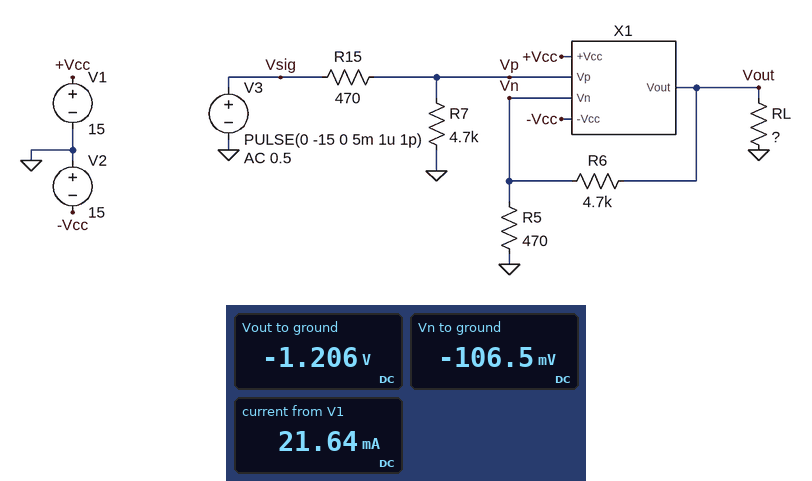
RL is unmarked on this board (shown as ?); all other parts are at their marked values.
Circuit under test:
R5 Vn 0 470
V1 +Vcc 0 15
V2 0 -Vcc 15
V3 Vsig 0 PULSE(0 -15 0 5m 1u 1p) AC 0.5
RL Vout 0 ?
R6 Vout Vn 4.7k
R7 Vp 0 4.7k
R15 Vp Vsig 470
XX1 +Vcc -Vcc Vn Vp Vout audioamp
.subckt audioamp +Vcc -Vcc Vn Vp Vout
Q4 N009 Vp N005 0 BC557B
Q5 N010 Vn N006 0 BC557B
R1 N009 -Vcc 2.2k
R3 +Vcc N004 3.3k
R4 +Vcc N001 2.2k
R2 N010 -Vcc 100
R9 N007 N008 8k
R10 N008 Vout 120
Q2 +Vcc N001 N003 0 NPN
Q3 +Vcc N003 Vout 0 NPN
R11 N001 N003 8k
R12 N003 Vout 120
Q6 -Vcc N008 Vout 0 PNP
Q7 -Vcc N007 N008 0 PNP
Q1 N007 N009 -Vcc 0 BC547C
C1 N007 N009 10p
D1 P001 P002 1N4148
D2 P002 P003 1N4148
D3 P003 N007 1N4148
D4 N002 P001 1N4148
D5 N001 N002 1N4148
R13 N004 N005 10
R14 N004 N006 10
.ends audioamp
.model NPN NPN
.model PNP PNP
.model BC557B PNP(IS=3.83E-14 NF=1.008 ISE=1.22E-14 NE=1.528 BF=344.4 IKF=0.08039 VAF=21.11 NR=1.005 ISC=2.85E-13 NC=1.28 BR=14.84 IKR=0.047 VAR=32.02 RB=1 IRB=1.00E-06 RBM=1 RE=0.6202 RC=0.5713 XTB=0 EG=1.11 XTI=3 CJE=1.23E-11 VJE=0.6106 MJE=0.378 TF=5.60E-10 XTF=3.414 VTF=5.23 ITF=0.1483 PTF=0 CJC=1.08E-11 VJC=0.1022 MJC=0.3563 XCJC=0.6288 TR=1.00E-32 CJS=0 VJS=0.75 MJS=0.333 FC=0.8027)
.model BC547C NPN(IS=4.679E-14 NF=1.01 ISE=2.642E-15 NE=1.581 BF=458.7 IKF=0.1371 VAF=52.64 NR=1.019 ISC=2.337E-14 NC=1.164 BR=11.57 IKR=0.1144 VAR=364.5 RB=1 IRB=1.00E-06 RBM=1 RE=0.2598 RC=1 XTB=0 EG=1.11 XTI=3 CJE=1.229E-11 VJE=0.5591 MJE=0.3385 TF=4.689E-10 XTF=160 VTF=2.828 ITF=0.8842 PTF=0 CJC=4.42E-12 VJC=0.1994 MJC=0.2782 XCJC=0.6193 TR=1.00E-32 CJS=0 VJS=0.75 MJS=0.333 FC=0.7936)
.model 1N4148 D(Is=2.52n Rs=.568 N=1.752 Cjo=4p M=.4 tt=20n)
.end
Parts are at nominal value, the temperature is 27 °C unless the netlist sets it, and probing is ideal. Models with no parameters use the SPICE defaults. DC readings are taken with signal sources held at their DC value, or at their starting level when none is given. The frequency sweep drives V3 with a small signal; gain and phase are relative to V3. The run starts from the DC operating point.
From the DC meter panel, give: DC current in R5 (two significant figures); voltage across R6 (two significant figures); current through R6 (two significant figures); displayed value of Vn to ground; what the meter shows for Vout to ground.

230 µA
1.1 V
230 µA
-106.5 mV
-1.206 V
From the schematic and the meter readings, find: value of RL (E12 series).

10 Ω
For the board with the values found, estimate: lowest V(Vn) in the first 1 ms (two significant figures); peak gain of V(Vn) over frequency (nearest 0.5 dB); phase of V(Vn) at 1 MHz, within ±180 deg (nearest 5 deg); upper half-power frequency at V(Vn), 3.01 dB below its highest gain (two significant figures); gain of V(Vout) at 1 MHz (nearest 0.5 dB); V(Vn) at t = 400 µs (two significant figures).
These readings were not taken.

-1.2 V
0 dB
-5 deg
11 MHz
20.0 dB
-1.2 V
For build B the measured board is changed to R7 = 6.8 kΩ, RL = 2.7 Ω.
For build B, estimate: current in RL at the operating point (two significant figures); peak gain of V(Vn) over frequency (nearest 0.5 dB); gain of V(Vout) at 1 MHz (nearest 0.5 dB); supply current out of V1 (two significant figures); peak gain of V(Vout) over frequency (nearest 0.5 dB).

450 mA
0.5 dB
20.5 dB
18 mA
22.5 dB
